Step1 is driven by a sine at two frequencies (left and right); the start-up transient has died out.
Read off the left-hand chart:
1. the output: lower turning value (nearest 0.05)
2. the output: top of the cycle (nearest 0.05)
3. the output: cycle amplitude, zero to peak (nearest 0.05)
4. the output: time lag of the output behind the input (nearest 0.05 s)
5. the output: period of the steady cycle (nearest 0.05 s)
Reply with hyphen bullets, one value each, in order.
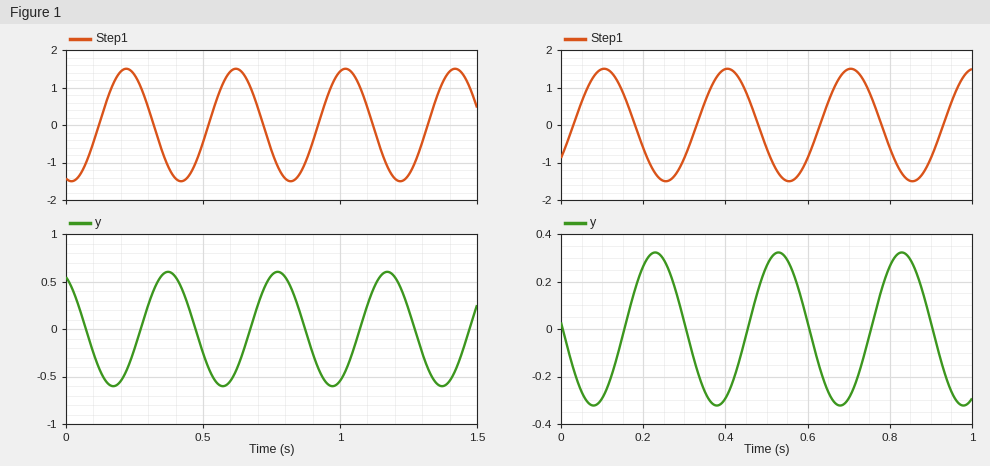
- -0.60
- 0.60
- 0.60
- 0.15 s
- 0.40 s
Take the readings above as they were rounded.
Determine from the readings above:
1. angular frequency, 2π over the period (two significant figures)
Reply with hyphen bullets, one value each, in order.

- 16 rad/s
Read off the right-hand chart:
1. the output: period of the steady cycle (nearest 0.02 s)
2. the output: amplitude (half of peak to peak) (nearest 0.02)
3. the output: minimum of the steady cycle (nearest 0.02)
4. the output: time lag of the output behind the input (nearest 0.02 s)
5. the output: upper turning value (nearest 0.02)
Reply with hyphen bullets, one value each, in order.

- 0.30 s
- 0.32
- -0.32
- 0.12 s
- 0.32
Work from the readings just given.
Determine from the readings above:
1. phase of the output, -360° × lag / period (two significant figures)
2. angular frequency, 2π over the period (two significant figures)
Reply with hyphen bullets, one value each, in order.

- -140°
- 21 rad/s
